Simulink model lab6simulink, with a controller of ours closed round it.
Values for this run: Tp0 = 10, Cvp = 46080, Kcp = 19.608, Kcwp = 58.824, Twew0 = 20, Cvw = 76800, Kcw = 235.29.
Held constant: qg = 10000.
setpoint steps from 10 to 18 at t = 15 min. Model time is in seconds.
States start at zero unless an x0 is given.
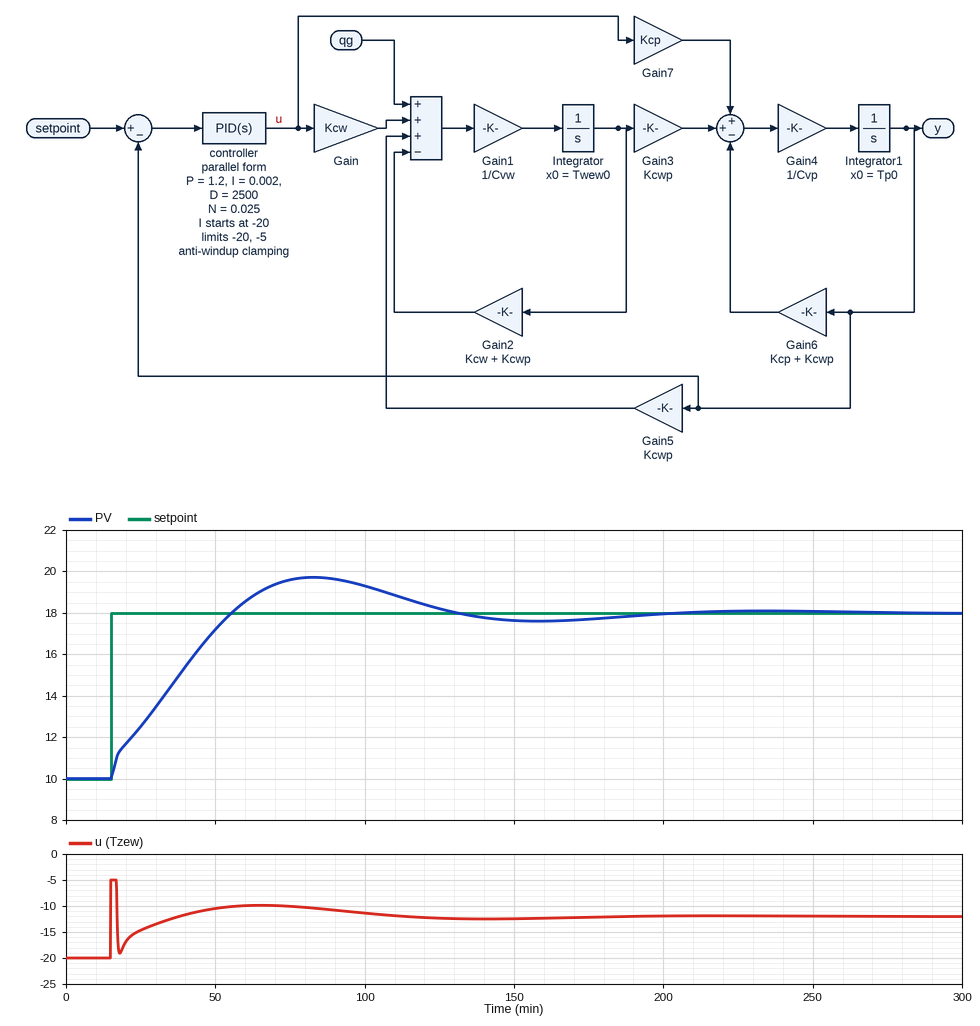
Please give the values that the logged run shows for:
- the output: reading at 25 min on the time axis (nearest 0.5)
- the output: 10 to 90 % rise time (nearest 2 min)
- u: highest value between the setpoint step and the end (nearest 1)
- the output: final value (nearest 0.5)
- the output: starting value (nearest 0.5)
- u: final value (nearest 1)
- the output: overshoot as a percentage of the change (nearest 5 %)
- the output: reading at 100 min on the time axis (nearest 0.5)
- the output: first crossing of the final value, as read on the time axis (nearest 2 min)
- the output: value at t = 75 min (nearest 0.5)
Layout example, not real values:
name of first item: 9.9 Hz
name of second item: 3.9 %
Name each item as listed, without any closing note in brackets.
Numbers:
the output: reading at 25 min on the time axis: 12.5
the output: 10 to 90 % rise time: 34 min
u: highest value between the setpoint step and the end: -5
the output: final value: 18.0
the output: starting value: 10.0
u: final value: -12
the output: overshoot as a percentage of the change: 20 %
the output: reading at 100 min on the time axis: 19.5
the output: first crossing of the final value, as read on the time axis: 56 min
the output: value at t = 75 min: 19.5
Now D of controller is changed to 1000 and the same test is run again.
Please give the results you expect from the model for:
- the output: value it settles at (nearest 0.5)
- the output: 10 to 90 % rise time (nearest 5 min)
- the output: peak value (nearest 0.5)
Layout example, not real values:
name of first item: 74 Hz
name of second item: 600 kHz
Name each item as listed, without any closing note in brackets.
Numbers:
the output: value it settles at: 18.0
the output: 10 to 90 % rise time: 25 min
the output: peak value: 19.0
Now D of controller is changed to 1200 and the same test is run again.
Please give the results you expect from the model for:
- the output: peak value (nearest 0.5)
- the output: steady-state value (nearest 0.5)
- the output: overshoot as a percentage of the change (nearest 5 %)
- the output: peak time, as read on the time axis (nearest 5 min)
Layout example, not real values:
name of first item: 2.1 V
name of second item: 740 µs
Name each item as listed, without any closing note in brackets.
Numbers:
the output: peak value: 19.0
the output: steady-state value: 18.0
the output: overshoot as a percentage of the change: 15 %
the output: peak time, as read on the time axis: 70 min
